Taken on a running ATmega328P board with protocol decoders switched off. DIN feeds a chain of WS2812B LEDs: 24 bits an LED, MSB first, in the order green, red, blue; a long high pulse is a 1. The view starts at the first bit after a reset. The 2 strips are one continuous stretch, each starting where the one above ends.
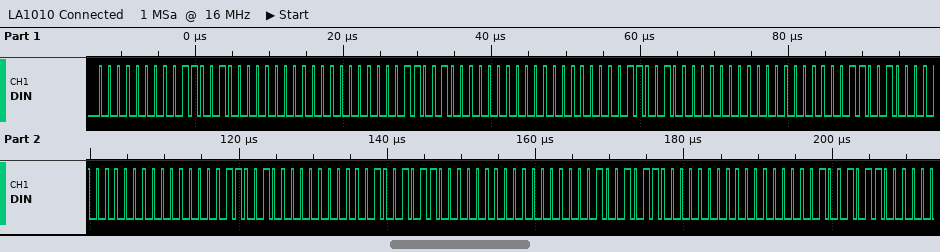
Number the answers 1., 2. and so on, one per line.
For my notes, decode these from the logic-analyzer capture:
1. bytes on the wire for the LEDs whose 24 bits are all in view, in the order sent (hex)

1. 00 64 00 00 64 00 00 64 00 00 64 00 00 64 00 4B 00 00 4B 00 00
